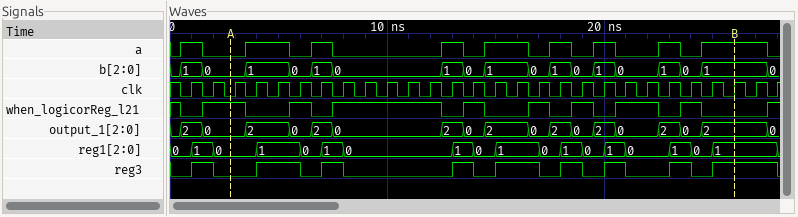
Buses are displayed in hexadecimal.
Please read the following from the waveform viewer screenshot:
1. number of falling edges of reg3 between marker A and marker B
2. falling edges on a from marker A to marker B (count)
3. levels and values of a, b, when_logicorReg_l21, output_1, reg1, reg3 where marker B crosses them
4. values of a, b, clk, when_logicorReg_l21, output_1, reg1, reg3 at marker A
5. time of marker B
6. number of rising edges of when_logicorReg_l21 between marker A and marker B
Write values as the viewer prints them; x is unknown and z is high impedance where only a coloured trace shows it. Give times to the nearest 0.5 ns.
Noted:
7
7
a=1, b=1, when_logicorReg_l21=0, output_1=2, reg1=1, reg3=1
a=0, b=0, clk=0, when_logicorReg_l21=1, output_1=0, reg1=0, reg3=0
26 ns
7
